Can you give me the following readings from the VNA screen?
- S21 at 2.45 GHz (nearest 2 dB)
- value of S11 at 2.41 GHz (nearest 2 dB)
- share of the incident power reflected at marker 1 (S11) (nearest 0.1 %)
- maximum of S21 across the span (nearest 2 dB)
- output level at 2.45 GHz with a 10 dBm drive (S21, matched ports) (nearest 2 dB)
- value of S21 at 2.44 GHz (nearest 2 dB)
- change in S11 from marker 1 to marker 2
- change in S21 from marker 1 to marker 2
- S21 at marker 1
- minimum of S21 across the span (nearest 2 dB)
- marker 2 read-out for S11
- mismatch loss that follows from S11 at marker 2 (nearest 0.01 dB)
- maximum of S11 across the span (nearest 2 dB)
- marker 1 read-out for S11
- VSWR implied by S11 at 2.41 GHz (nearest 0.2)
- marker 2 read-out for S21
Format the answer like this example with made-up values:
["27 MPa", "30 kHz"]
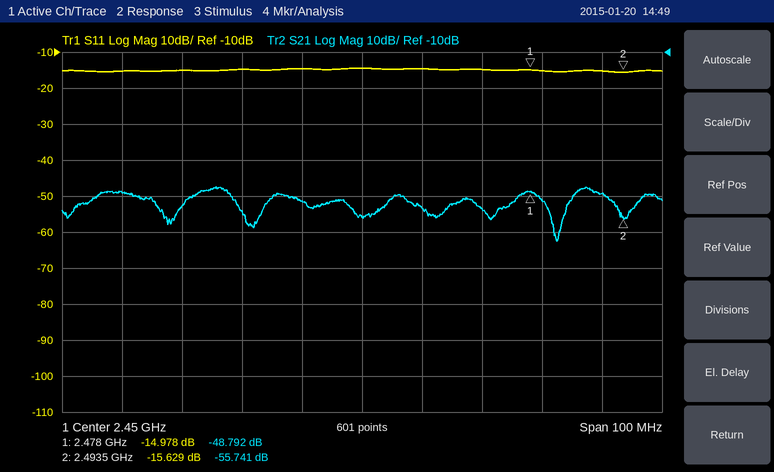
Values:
["-56 dB", "-16 dB", "3.2 %", "-48 dB", "-46 dBm", "-52 dB", "-0.651 dB", "-6.949 dB", "-48.792 dB", "-62 dB", "-15.629 dB", "0.12 dB", "-14 dB", "-14.978 dB", "1.4", "-55.741 dB"]
